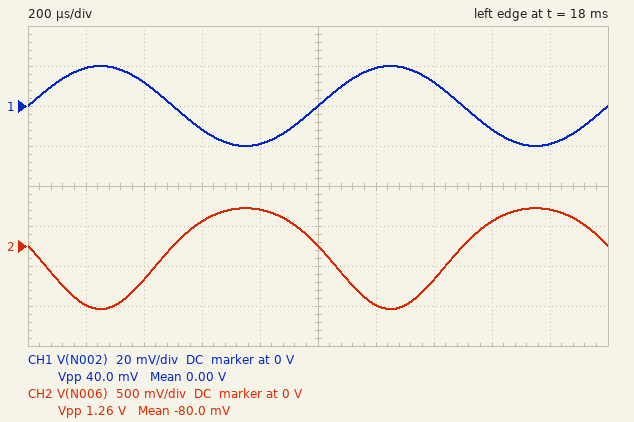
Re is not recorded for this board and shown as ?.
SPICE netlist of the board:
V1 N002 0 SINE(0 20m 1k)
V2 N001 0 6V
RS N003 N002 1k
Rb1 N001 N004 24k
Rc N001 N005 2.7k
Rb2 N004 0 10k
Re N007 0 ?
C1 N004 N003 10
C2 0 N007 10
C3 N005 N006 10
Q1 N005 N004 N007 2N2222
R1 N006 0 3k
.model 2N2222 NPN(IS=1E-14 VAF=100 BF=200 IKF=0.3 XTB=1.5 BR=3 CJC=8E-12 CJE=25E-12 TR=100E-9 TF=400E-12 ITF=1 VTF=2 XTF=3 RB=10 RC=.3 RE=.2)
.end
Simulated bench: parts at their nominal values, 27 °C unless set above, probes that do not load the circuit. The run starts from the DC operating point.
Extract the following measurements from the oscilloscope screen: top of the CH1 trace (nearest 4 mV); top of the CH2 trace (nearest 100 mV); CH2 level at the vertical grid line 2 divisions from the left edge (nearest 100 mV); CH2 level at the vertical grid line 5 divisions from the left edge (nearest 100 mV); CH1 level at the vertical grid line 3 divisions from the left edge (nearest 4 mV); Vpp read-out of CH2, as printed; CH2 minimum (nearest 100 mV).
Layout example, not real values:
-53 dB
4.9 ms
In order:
20 mV
500 mV
-400 mV
0 V
-12 mV
1.26 V
-800 mV
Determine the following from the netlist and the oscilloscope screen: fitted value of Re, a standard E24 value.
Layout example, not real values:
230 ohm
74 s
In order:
1.5 kΩ
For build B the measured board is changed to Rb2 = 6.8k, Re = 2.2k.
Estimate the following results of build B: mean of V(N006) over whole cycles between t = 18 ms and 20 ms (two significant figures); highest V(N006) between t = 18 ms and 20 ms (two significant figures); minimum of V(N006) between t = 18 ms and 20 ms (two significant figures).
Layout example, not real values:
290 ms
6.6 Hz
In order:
-40 mV
210 mV
-370 mV
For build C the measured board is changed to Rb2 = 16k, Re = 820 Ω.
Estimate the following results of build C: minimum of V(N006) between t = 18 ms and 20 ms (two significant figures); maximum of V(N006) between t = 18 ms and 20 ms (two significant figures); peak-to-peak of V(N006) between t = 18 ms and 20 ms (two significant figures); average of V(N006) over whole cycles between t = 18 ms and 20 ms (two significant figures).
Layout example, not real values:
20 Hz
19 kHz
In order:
-13 mV
30 mV
43 mV
4.0 mV
